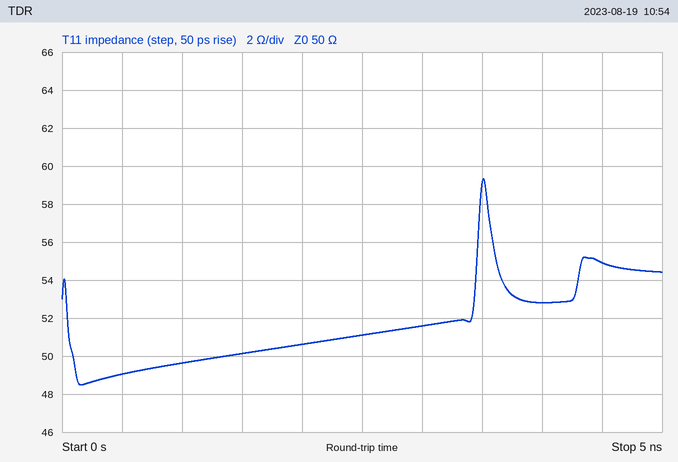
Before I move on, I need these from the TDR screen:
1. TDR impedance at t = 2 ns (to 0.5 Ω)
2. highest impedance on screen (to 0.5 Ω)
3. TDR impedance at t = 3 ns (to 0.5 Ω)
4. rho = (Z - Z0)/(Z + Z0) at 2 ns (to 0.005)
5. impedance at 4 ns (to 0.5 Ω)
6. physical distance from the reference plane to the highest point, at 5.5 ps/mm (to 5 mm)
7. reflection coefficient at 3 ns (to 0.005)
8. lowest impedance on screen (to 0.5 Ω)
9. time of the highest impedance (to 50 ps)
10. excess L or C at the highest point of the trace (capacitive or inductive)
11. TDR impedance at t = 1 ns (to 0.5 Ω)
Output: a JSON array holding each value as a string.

["50.5 Ω", "59.5 Ω", "51.5 Ω", "+0.005", "53.0 Ω", "320 mm", "+0.015", "48.5 Ω", "3.50 ns", "inductive", "49.5 Ω"]
